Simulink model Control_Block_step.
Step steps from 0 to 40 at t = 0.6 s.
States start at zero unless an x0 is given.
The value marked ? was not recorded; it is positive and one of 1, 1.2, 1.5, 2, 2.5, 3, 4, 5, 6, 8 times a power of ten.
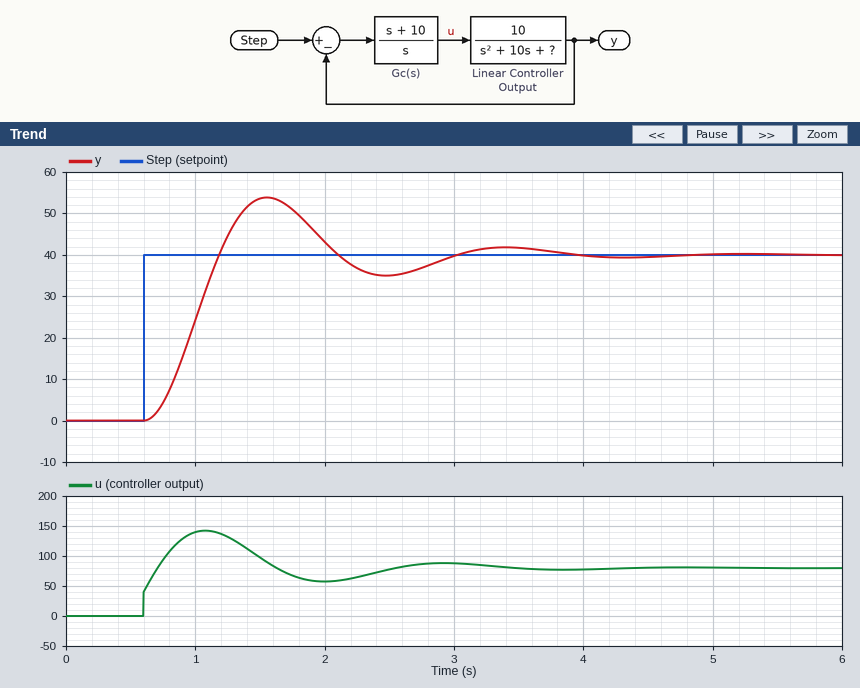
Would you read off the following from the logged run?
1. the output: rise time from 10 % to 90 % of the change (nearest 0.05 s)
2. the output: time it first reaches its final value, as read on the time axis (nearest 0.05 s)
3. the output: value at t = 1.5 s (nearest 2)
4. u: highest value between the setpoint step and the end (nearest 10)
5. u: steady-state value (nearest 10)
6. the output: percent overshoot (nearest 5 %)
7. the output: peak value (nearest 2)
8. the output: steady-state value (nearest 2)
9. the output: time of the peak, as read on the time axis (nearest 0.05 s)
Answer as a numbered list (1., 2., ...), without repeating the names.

1. 0.40 s
2. 1.20 s
3. 54
4. 140
5. 80
6. 35 %
7. 54
8. 40
9. 1.55 s
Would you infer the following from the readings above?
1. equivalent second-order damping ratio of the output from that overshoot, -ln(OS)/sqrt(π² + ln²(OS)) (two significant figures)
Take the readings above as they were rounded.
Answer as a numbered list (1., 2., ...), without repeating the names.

1. 0.32
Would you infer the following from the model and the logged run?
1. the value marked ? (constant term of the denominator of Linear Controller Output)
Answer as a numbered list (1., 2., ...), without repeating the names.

1. 20
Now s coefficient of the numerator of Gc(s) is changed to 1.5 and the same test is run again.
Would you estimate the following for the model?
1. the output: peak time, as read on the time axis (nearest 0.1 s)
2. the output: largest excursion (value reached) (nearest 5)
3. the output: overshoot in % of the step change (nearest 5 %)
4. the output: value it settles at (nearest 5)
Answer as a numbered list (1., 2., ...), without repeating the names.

1. 1.5 s
2. 50
3. 25 %
4. 40
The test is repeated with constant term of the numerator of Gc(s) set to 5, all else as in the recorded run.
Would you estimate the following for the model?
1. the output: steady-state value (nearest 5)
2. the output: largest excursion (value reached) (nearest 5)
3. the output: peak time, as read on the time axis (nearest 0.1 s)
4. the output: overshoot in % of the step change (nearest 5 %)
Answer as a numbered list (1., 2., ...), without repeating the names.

1. 40
2. 45
3. 2.0 s
4. 10 %
